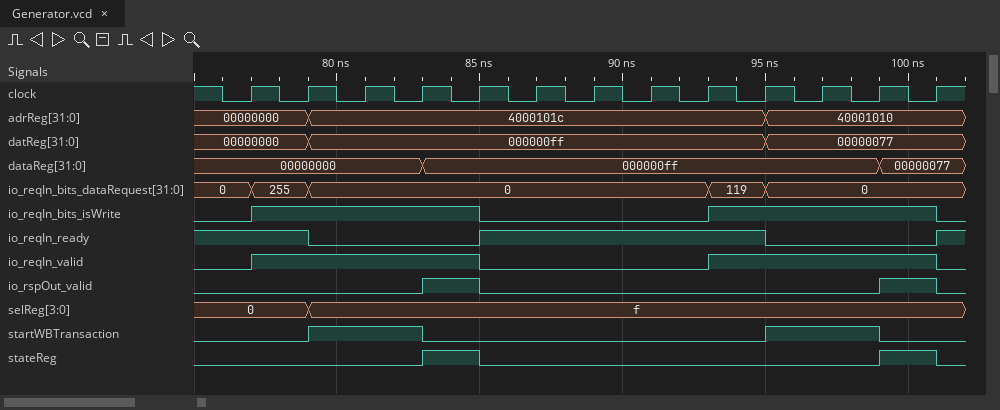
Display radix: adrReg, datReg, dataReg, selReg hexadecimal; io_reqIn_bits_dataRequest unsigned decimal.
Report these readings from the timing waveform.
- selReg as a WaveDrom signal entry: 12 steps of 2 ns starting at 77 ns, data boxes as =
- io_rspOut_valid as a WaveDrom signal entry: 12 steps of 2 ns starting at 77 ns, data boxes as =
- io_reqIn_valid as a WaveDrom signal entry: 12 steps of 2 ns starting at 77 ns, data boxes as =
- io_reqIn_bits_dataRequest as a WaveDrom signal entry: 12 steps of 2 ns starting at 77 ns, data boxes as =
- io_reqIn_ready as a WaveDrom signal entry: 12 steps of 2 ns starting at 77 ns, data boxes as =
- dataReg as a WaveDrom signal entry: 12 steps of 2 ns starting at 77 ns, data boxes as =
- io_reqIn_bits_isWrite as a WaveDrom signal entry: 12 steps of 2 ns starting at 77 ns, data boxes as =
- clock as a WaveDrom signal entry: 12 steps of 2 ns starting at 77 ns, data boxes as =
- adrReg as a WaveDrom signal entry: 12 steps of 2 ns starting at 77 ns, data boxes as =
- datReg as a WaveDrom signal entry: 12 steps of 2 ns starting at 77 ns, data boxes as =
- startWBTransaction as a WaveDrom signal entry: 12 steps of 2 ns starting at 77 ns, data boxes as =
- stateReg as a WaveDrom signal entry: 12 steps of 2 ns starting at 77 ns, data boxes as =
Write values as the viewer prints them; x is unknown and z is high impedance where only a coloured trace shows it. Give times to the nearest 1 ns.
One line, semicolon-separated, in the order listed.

{name: 'selReg', wave: '==..........', data: '0 f'}; {name: 'io_rspOut_valid', wave: '0..10......1'}; {name: 'io_reqIn_valid', wave: '1...0...1...'}; {name: 'io_reqIn_bits_dataRequest', wave: '==......==..', data: '255 0 119 0'}; {name: 'io_reqIn_ready', wave: '10..1....0..'}; {name: 'dataReg', wave: '=..=.......=', data: '00000000 000000ff 00000077'}; {name: 'io_reqIn_bits_isWrite', wave: '1...0...1...'}; {name: 'clock', wave: 'p...........'}; {name: 'adrReg', wave: '==.......=..', data: '00000000 4000101c 40001010'}; {name: 'datReg', wave: '==.......=..', data: '00000000 000000ff 00000077'}; {name: 'startWBTransaction', wave: '01.0.....1.0'}; {name: 'stateReg', wave: '0..10......1'}
